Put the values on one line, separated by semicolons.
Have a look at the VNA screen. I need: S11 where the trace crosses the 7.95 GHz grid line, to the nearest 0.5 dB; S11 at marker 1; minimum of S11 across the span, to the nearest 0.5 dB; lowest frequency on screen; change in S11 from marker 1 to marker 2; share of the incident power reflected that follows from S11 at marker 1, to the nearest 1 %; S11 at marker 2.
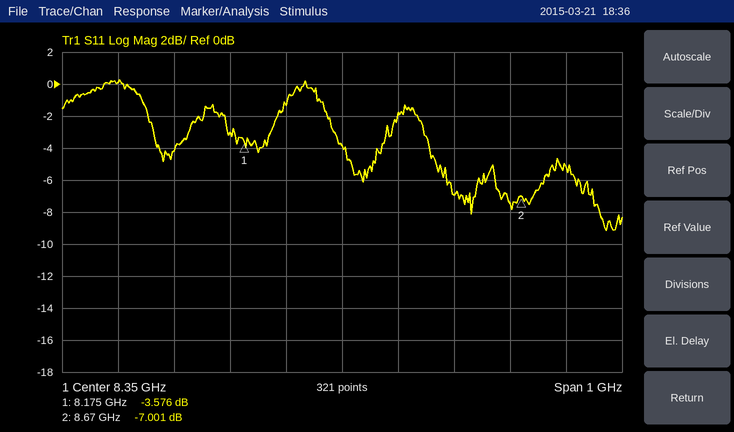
0.0 dB; -3.576 dB; -9.0 dB; 7.85 GHz; -3.425 dB; 44 %; -7.001 dB
